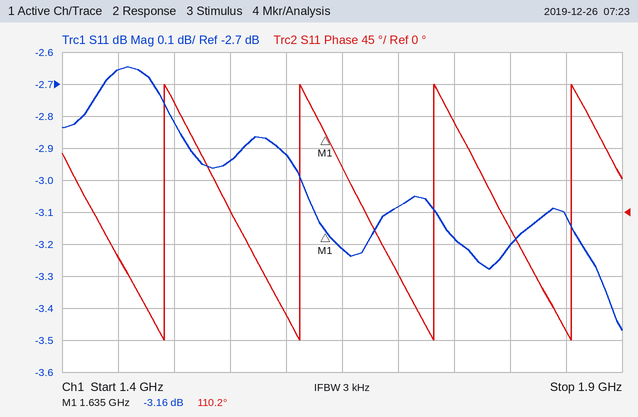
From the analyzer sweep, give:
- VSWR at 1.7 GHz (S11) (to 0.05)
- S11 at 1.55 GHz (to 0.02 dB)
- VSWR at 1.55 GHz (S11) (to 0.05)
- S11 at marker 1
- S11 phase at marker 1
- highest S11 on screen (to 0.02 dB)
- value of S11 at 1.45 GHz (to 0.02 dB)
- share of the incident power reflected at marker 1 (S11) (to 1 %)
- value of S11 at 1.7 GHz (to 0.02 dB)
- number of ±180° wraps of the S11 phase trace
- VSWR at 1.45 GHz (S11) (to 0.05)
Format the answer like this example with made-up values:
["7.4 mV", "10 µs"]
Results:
["5.70", "-2.94 dB", "5.95", "-3.16 dB", "110.2°", "-2.64 dB", "-2.66 dB", "48 %", "-3.08 dB", "4", "6.60"]
